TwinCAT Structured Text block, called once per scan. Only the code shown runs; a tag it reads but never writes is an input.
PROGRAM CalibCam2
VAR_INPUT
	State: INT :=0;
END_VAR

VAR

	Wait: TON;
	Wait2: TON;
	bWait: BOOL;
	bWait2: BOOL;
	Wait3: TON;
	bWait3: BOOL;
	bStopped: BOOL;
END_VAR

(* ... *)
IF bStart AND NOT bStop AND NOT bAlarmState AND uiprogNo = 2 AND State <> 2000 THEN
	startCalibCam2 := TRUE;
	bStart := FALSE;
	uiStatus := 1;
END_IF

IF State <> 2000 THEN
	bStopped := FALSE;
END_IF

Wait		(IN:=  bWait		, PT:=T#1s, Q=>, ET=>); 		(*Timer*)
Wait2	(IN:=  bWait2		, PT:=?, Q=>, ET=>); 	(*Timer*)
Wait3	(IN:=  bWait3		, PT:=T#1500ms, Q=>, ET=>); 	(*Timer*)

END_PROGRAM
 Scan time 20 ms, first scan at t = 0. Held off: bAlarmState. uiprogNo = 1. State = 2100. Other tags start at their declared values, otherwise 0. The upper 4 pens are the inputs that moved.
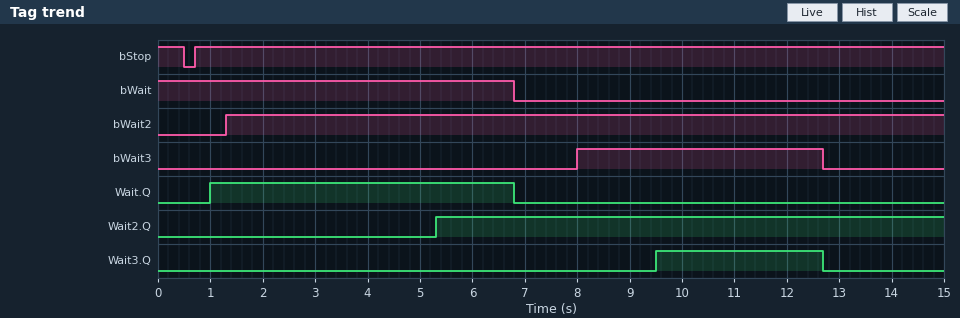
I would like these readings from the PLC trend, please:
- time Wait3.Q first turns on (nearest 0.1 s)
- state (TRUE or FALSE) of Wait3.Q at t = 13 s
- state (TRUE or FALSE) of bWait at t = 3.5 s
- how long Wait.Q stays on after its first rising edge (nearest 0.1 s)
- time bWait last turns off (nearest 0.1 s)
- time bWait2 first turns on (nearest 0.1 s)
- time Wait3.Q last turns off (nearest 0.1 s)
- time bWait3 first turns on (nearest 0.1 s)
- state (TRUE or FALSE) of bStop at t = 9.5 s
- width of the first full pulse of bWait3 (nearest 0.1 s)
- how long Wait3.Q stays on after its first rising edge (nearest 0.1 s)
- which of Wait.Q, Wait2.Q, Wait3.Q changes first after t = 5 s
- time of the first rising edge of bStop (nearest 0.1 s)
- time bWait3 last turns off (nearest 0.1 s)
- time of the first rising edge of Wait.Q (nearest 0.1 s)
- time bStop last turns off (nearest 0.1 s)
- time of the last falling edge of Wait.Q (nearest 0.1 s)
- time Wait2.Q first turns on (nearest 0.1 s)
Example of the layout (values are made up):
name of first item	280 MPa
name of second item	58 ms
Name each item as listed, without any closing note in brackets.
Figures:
time Wait3.Q first turns on	9.5 s
state (TRUE or FALSE) of Wait3.Q at t = 13 s	FALSE
state (TRUE or FALSE) of bWait at t = 3.5 s	TRUE
how long Wait.Q stays on after its first rising edge	5.8 s
time bWait last turns off	6.8 s
time bWait2 first turns on	1.3 s
time Wait3.Q last turns off	12.7 s
time bWait3 first turns on	8.0 s
state (TRUE or FALSE) of bStop at t = 9.5 s	TRUE
width of the first full pulse of bWait3	4.7 s
how long Wait3.Q stays on after its first rising edge	3.2 s
which of Wait.Q, Wait2.Q, Wait3.Q changes first after t = 5 s	Wait2.Q
time of the first rising edge of bStop	0.7 s
time bWait3 last turns off	12.7 s
time of the first rising edge of Wait.Q	1.0 s
time bStop last turns off	0.5 s
time of the last falling edge of Wait.Q	6.8 s
time Wait2.Q first turns on	5.3 s
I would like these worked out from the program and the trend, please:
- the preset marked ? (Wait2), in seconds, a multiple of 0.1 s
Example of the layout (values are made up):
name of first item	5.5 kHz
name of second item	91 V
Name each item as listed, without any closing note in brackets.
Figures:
the preset marked ? (Wait2), in seconds, a multiple of 0.1 s	4.0 s
